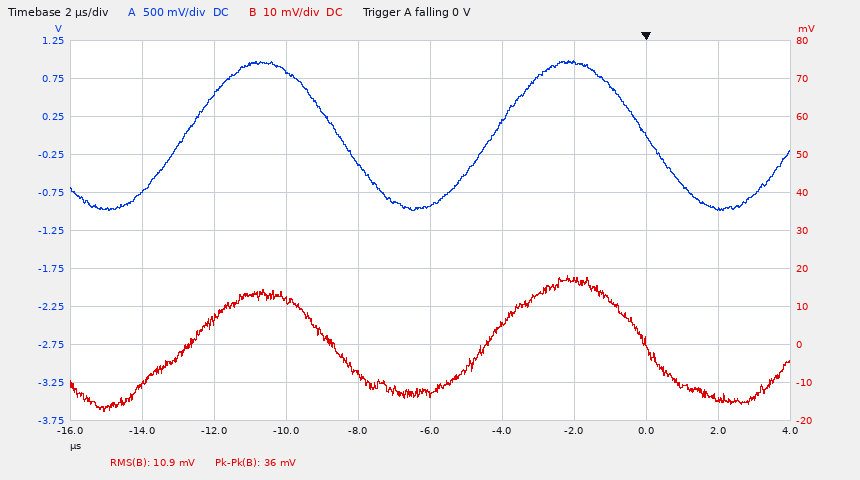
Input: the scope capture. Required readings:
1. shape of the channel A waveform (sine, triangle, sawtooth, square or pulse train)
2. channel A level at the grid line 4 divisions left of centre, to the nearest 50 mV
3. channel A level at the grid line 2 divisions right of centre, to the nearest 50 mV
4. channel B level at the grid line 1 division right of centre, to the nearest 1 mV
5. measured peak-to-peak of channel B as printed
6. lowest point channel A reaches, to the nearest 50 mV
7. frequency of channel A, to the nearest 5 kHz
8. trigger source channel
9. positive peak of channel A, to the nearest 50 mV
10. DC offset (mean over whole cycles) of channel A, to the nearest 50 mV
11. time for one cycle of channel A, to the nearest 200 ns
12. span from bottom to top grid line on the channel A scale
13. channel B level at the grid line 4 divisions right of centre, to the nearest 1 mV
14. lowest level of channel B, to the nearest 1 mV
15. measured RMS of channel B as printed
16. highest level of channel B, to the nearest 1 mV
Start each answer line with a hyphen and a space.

- sine
- -750 mV
- 950 mV
- 5 mV
- 36 mV
- -1.00 V
- 115 kHz
- channel A
- 1.00 V
- 0 mV
- 8.6 µs
- 5 V
- -15 mV
- -18 mV
- 10.9 mV
- 18 mV
